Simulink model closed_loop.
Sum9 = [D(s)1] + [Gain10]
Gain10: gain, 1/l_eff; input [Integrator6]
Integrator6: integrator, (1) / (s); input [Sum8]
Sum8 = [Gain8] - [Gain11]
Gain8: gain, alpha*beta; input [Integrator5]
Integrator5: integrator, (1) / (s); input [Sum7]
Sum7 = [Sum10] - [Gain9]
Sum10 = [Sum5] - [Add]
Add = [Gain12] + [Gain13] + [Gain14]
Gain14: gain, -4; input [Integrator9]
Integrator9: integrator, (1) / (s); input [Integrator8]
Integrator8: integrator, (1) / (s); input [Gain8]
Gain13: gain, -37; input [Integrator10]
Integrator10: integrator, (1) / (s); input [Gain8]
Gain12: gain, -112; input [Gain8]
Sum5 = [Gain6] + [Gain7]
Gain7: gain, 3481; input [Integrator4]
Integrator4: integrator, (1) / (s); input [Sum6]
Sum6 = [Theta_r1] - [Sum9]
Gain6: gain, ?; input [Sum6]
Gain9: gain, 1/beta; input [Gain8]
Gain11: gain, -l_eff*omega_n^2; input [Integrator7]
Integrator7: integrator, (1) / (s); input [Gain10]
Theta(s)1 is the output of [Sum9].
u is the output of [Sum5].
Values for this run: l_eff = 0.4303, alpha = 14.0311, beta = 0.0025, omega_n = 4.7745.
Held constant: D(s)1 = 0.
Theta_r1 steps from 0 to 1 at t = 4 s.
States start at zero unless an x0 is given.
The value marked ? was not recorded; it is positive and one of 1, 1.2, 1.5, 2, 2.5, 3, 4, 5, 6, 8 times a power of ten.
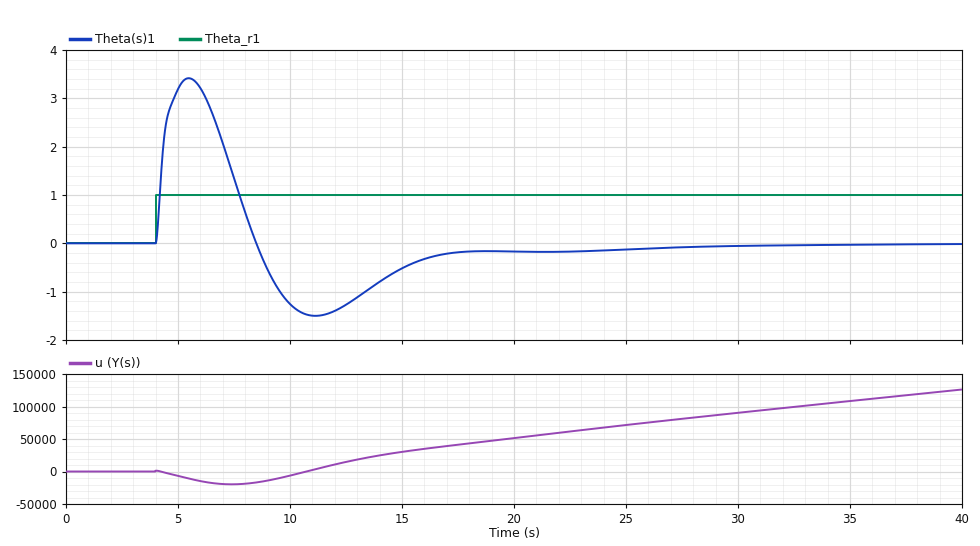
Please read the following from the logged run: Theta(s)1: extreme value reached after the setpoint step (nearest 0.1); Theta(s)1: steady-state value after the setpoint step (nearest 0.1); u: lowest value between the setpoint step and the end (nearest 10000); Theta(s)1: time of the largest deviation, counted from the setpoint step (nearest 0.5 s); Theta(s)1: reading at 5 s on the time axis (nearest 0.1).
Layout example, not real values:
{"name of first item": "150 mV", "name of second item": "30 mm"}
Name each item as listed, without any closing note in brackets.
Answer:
{"Theta(s)1: extreme value reached after the setpoint step": "3.4", "Theta(s)1: steady-state value after the setpoint step": "0.0", "u: lowest value between the setpoint step and the end": "-20000", "Theta(s)1: time of the largest deviation, counted from the setpoint step": "1.5 s", "Theta(s)1: reading at 5 s on the time axis": "3.2"}
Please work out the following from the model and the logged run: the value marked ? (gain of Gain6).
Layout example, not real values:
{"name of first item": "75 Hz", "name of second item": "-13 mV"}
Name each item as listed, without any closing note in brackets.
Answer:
{"the value marked ?": "1200"}
